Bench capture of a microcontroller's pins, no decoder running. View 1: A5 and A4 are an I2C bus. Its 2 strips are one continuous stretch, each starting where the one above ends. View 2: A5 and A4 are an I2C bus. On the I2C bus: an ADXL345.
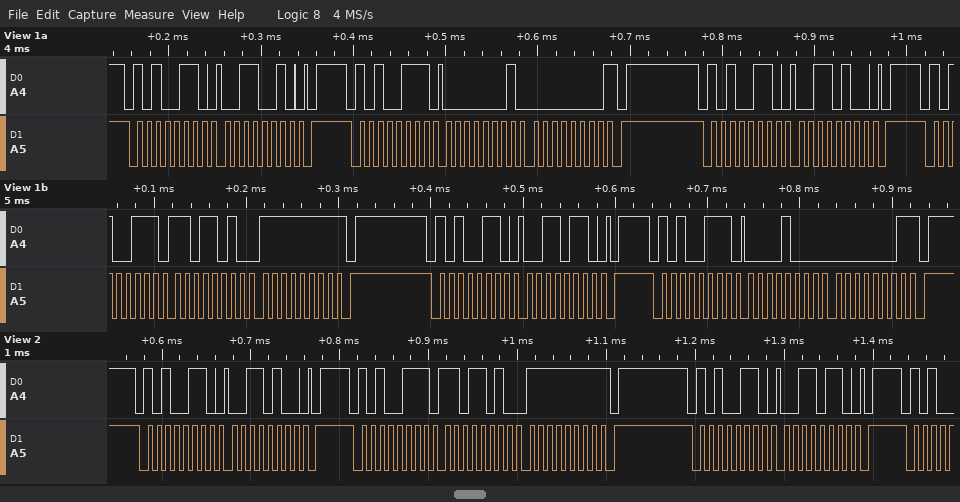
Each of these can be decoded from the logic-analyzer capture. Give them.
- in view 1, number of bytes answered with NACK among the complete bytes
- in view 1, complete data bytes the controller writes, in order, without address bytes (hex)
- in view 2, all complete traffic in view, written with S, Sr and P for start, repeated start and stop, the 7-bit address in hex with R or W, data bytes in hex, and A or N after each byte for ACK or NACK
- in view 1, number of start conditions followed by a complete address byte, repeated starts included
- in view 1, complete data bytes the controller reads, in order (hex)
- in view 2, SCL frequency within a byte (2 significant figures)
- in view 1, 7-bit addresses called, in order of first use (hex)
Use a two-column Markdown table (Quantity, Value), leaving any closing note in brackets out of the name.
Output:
| Quantity | Value |
|---|---|
| in view 1, number of bytes answered with NACK among the complete bytes | 3 |
| in view 1, complete data bytes the controller writes, in order, without address bytes | 32 34 36 |
| in view 2, all complete traffic in view, written with S, Sr and P for start, repeated start and stop, the 7-bit address in hex with R or W, data bytes in hex, and A or N after each byte for ACK or NACK | S 53W A 34 A P S 53R A DA A FF N P S 53W A 36 A P |
| in view 1, number of start conditions followed by a complete address byte, repeated starts included | 6 |
| in view 1, complete data bytes the controller reads, in order | 01 00 DA FF 08 01 |
| in view 2, SCL frequency within a byte | 100 kHz |
| in view 1, 7-bit addresses called, in order of first use | 0x53 |
